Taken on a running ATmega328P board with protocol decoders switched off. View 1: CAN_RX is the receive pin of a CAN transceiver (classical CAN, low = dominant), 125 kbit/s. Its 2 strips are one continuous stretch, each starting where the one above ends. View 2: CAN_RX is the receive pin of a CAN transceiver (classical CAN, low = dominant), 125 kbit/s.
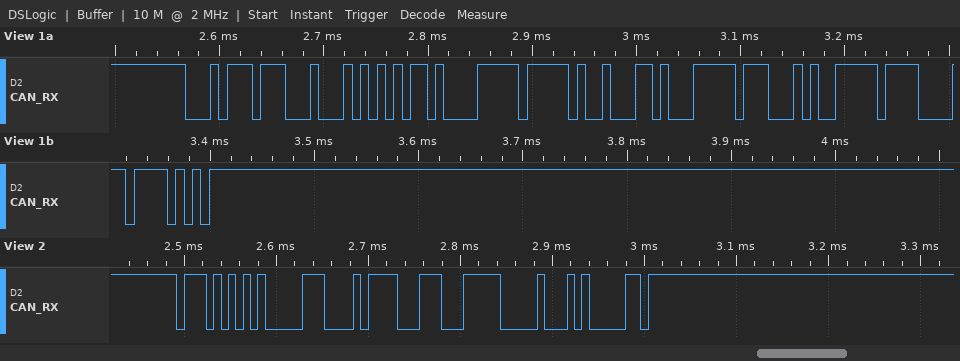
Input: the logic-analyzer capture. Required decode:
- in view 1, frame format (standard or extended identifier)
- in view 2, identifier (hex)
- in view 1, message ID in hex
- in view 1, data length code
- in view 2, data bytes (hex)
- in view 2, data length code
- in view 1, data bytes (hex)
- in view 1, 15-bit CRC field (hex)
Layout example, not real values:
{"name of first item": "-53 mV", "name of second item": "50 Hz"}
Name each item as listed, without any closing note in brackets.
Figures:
{"in view 1, frame format": "standard", "in view 2, identifier": "0x755", "in view 1, message ID in hex": "0x177", "in view 1, data length code": "8", "in view 2, data bytes": "0B C7 1F", "in view 2, data length code": "3", "in view 1, data bytes": "AA D0 FF E4 68 FF 14 FF", "in view 1, 15-bit CRC field": "0x437A"}
